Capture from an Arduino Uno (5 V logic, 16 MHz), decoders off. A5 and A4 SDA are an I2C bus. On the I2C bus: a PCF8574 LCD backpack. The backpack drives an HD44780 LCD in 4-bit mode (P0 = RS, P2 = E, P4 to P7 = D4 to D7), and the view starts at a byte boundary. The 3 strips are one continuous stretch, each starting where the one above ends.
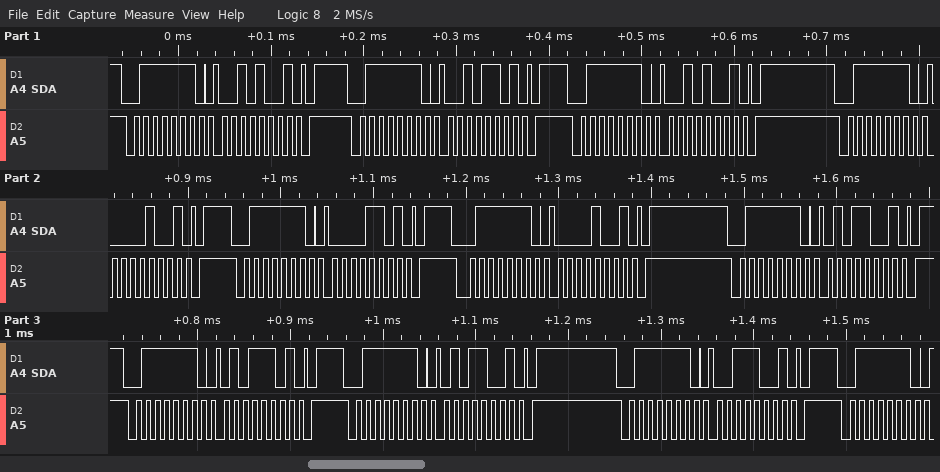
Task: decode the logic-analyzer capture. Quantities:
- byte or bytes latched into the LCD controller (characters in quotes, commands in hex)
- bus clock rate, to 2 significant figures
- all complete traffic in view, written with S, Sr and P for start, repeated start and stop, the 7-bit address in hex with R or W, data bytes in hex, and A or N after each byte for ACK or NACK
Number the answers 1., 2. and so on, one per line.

1. ' '
2. 100 kHz
3. S 3FW A 29 A P S 3FW A 2D A P S 3FW A 29 A P S 3FW A 09 A P S 3FW A 0D A P S 3FW A 09 A P S 3FW A 59 A P S 3FW A 5D A P S 3FW A 59 A P S 3FW A 39 A P S 3FW A
